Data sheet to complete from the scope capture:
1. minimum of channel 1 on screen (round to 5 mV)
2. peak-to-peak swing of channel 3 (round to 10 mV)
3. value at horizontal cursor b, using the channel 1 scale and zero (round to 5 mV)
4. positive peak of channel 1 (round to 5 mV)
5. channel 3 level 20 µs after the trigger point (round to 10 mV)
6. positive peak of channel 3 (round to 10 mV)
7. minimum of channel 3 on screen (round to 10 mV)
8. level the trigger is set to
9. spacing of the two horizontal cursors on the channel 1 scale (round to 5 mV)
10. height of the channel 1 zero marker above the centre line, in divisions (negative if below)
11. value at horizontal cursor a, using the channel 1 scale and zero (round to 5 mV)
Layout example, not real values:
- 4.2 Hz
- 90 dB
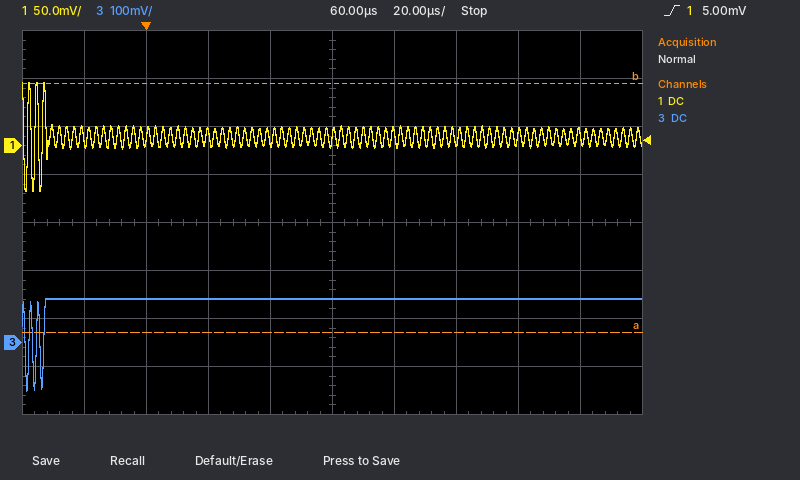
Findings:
- -45 mV
- 190 mV
- 65 mV
- 65 mV
- 90 mV
- 90 mV
- -100 mV
- 5.00 mV
- 260 mV
- +1.6 div
- -195 mV
